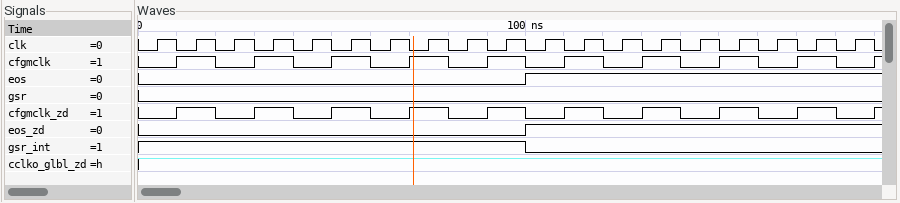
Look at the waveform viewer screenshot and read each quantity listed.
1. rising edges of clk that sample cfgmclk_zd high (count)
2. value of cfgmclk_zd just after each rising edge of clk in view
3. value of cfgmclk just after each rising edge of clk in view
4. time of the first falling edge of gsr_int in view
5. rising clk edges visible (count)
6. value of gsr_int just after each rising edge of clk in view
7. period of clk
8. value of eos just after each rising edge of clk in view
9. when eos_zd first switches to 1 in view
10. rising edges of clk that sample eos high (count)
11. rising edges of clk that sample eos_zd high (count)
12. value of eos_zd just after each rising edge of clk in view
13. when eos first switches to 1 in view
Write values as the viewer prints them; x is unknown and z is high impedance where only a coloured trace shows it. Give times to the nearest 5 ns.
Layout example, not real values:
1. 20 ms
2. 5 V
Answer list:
1. 9
2. 0 1 0 1 0 1 0 1 0 1 0 1 0 1 0 1 0 1 0
3. 0 1 0 1 0 1 0 1 0 1 0 1 0 1 0 1 0 1 0
4. 100 ns
5. 19
6. 1 1 1 1 1 1 1 1 1 1 0 0 0 0 0 0 0 0 0
7. 10 ns
8. 0 0 0 0 0 0 0 0 0 0 1 1 1 1 1 1 1 1 1
9. 100 ns
10. 9
11. 9
12. 0 0 0 0 0 0 0 0 0 0 1 1 1 1 1 1 1 1 1
13. 100 ns
